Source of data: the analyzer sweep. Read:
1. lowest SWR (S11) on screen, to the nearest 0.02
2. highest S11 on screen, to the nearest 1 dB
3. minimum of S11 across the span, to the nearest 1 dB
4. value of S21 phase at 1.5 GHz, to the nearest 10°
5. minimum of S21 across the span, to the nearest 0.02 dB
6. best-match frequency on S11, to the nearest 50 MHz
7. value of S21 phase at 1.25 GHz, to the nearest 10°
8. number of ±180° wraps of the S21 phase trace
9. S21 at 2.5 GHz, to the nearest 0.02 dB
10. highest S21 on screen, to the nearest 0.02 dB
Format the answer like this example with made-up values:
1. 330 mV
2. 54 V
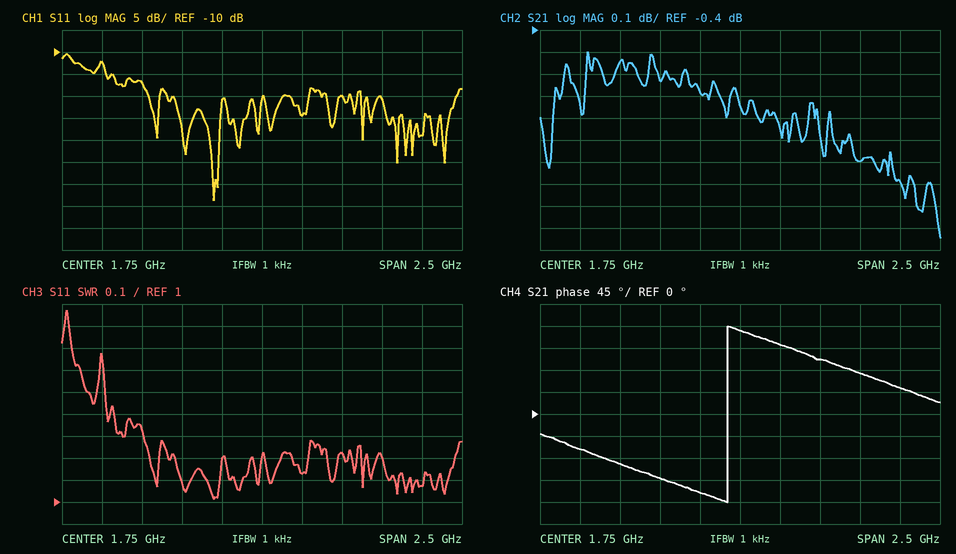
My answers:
1. 1.02
2. -10 dB
3. -44 dB
4. -160°
5. -1.34 dB
6. 1.45 GHz
7. -130°
8. 1
9. -1.00 dB
10. -0.50 dB
